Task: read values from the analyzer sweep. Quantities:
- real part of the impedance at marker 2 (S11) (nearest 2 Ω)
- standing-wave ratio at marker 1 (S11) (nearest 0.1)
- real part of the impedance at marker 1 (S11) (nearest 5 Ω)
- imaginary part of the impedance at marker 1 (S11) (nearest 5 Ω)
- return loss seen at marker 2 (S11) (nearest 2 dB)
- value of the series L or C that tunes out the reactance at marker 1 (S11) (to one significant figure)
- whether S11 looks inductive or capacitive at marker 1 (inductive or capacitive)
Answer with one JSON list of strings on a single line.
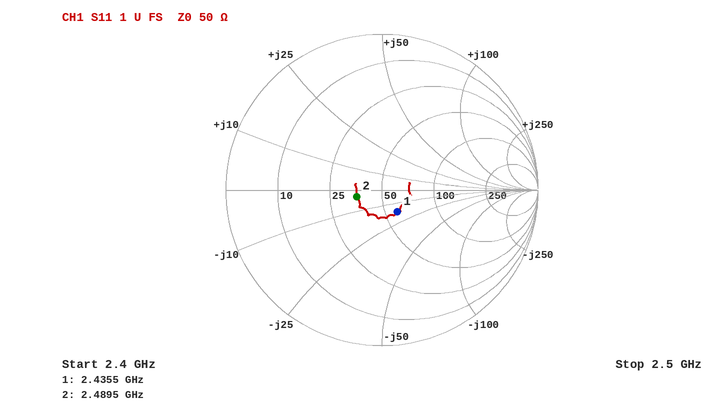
["36 Ω", "1.4", "60 Ω", "-15 Ω", "16 dB", "1 nH", "capacitive"]
